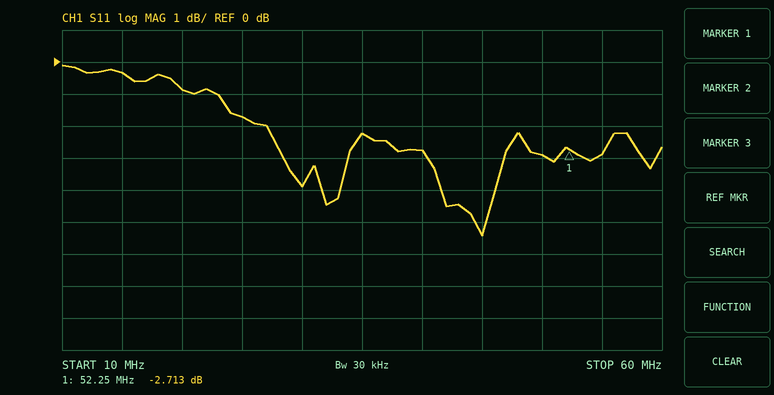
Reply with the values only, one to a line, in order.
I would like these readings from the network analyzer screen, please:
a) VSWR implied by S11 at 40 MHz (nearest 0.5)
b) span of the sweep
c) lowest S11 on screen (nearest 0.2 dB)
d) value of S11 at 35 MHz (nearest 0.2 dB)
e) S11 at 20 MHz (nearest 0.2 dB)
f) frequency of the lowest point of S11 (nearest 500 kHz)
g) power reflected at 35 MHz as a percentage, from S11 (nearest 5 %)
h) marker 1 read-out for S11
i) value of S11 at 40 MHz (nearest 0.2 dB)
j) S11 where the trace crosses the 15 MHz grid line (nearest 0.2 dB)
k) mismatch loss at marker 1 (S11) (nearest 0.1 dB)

6.5
50 MHz
-5.4 dB
-2.2 dB
-0.8 dB
45.0 MHz
60 %
-2.713 dB
-2.8 dB
-0.4 dB
3.3 dB
